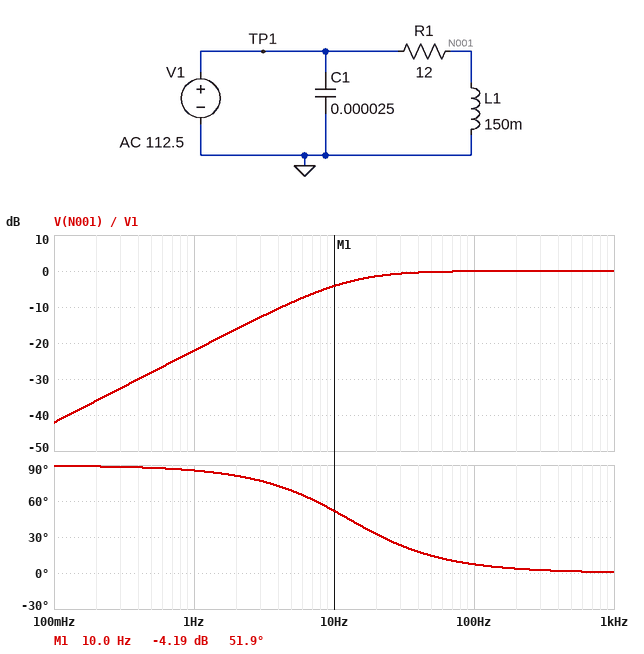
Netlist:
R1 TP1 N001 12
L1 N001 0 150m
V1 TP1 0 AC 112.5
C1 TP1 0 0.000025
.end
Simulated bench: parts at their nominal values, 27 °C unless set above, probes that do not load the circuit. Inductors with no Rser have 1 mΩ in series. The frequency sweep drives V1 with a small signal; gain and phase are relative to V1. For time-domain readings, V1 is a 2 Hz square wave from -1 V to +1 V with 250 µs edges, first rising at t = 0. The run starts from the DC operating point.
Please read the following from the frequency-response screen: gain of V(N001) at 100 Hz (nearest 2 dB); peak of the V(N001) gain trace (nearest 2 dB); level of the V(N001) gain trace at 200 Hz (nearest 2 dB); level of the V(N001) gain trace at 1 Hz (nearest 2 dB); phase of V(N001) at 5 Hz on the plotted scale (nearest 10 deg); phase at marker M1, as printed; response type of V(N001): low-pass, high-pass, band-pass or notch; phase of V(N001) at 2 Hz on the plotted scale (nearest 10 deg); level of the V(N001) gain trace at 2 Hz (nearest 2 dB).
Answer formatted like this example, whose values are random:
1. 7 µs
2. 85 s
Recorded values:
1. 0 dB
2. 0 dB
3. 0 dB
4. -22 dB
5. 70 deg
6. 51.9 deg
7. high-pass
8. 80 deg
9. -16 dB
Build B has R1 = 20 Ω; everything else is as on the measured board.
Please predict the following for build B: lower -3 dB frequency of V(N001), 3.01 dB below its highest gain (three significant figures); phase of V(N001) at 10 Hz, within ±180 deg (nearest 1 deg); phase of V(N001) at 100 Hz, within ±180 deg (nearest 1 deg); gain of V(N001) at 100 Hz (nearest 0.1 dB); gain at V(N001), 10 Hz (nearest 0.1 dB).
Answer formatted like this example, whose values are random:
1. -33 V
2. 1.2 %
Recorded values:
1. 21.2 Hz
2. 65 deg
3. 12 deg
4. -0.2 dB
5. -7.4 dB
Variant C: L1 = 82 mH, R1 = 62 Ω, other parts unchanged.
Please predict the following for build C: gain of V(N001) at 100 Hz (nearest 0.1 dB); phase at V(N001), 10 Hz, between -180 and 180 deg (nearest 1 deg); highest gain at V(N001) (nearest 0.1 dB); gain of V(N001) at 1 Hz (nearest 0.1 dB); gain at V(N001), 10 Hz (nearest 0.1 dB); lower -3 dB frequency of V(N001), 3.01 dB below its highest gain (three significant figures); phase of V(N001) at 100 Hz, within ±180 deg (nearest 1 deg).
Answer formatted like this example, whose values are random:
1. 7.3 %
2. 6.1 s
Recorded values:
1. -3.9 dB
2. 85 deg
3. 0 dB
4. -41.6 dB
5. -21.6 dB
6. 120 Hz
7. 50 deg
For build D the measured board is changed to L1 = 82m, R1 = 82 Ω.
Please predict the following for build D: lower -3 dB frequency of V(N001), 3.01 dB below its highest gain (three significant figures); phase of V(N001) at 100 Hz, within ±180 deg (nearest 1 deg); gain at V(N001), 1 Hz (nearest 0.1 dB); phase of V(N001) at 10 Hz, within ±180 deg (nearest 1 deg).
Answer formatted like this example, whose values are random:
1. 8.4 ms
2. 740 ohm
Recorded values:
1. 159 Hz
2. 58 deg
3. -44.0 dB
4. 86 deg
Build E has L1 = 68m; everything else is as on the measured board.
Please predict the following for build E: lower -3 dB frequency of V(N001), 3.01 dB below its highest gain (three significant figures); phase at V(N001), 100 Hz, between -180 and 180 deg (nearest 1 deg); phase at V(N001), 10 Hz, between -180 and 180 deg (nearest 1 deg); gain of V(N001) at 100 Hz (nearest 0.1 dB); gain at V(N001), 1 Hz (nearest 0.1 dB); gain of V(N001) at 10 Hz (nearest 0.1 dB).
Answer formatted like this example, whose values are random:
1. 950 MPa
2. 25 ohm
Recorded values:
1. 28.1 Hz
2. 16 deg
3. 70 deg
4. -0.3 dB
5. -29.0 dB
6. -9.5 dB
